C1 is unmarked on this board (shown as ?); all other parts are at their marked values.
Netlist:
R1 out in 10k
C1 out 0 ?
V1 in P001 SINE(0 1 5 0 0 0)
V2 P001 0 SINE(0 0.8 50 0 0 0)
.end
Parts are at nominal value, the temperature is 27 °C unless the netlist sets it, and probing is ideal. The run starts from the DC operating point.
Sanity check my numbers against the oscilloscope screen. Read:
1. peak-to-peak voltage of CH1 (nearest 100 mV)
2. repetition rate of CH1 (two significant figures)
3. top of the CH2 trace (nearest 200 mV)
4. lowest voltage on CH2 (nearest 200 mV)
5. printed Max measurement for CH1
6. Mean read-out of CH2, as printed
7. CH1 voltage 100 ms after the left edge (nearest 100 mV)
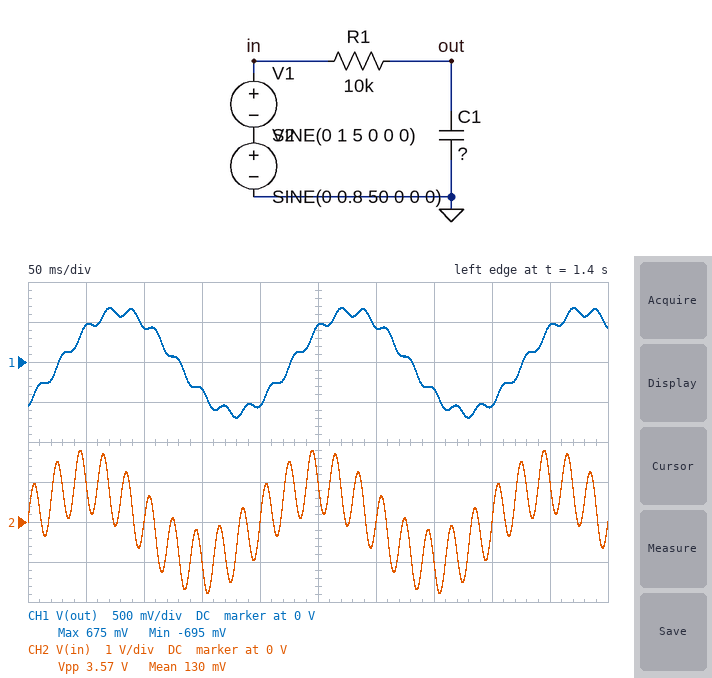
1.4 V
5.0 Hz
1.8 V
-1.8 V
675 mV
130 mV
400 mV
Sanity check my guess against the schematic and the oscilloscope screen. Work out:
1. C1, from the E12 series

3.9 µF
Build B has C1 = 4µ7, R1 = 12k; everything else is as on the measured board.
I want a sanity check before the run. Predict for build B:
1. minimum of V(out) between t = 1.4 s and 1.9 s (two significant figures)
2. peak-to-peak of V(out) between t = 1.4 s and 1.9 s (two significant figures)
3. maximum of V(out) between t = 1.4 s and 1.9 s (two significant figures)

-530 mV
1.1 V
530 mV
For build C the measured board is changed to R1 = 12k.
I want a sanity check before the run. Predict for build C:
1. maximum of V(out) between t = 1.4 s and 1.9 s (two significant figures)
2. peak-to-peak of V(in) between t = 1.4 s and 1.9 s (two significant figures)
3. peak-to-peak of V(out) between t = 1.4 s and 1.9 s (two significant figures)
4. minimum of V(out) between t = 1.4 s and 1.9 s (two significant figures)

600 mV
3.6 V
1.2 V
-620 mV
